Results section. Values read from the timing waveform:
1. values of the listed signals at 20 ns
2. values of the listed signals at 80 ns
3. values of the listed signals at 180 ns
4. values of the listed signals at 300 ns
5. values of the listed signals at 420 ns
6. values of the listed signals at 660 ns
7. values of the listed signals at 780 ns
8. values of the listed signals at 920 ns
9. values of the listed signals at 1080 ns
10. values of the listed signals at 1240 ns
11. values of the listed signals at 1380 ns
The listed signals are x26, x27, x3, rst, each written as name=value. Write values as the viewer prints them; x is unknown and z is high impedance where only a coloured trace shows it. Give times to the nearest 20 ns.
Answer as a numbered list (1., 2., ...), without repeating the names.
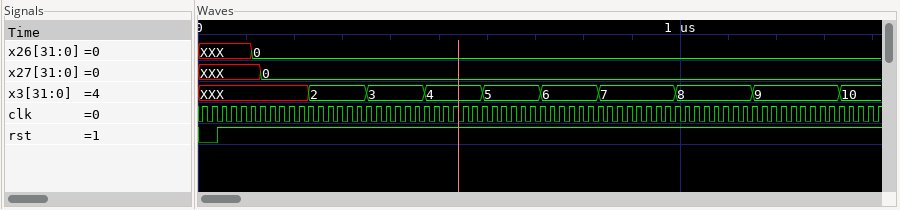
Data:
1. x26=XXX, x27=XXX, x3=XXX, rst=0
2. x26=XXX, x27=XXX, x3=XXX, rst=1
3. x26=0, x27=0, x3=XXX, rst=1
4. x26=0, x27=0, x3=2, rst=1
5. x26=0, x27=0, x3=3, rst=1
6. x26=0, x27=0, x3=5, rst=1
7. x26=0, x27=0, x3=6, rst=1
8. x26=0, x27=0, x3=7, rst=1
9. x26=0, x27=0, x3=8, rst=1
10. x26=0, x27=0, x3=9, rst=1
11. x26=0, x27=0, x3=10, rst=1
